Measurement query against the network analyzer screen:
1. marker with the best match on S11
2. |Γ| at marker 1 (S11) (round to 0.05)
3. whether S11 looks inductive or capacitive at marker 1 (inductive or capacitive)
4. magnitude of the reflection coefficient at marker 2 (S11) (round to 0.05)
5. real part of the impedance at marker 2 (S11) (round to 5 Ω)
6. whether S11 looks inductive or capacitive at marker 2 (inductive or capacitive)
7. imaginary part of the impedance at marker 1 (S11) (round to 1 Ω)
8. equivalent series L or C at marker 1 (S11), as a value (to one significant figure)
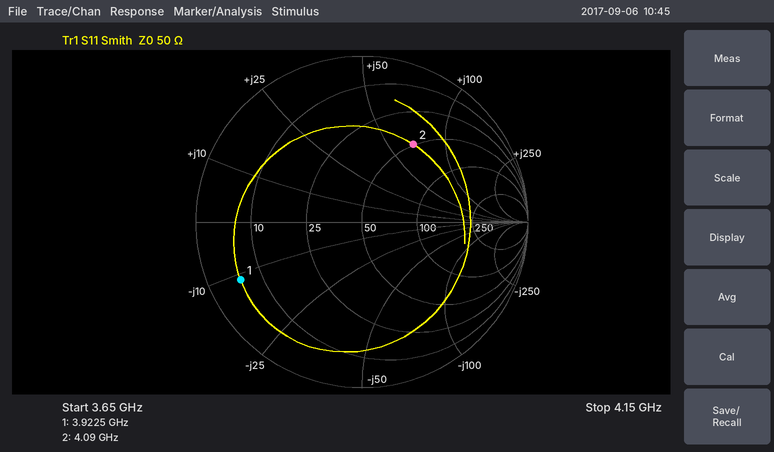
marker 2
0.80
capacitive
0.55
50 Ω
inductive
-11 Ω
4 pF
